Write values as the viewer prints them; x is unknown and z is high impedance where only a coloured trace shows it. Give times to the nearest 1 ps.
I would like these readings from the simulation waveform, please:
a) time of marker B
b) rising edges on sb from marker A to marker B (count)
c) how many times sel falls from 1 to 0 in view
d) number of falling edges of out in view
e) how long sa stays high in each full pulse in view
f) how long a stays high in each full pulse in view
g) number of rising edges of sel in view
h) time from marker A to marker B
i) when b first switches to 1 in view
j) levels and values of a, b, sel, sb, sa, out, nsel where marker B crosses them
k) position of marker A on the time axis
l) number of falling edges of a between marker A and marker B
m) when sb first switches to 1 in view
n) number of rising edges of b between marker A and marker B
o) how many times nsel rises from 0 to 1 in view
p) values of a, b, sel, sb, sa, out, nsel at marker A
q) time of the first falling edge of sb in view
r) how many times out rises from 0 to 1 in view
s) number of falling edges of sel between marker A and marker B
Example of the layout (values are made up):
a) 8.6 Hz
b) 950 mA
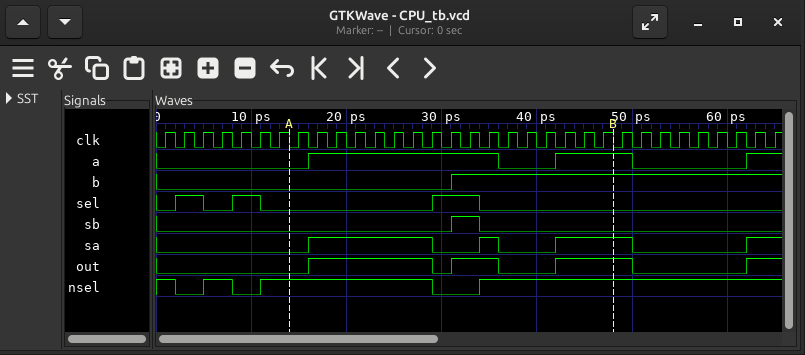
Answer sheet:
a) 48 ps
b) 1
c) 3
d) 3
e) 13 ps, 2 ps, 8 ps
f) 20 ps, 8 ps
g) 3
h) 34 ps
i) 31 ps
j) a=1, b=1, sel=0, sb=0, sa=1, out=1, nsel=1
k) 14 ps
l) 1
m) 31 ps
n) 1
o) 3
p) a=0, b=0, sel=0, sb=0, sa=0, out=0, nsel=1
q) 34 ps
r) 4
s) 1
